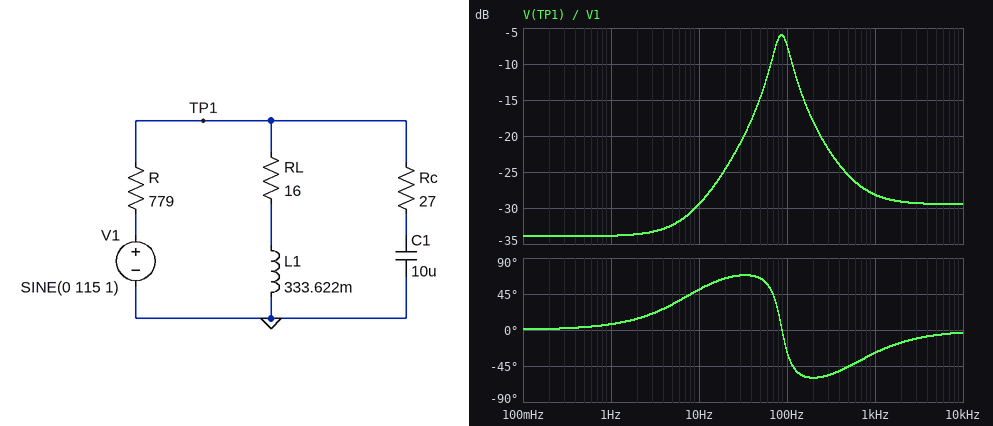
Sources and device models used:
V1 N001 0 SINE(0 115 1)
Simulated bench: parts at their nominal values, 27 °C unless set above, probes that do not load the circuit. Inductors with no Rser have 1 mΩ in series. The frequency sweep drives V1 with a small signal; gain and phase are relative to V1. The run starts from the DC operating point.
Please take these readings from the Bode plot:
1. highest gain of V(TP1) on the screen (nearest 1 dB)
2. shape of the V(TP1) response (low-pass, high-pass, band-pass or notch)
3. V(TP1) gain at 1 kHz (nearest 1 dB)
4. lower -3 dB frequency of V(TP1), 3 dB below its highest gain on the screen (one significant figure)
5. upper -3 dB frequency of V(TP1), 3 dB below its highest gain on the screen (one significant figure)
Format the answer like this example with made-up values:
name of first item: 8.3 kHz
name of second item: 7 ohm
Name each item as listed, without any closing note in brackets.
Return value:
highest gain of V(TP1) on the screen: -6 dB
shape of the V(TP1) response: band-pass
V(TP1) gain at 1 kHz: -28 dB
lower -3 dB frequency of V(TP1), 3 dB below its highest gain on the screen: 70 Hz
upper -3 dB frequency of V(TP1), 3 dB below its highest gain on the screen: 100 Hz
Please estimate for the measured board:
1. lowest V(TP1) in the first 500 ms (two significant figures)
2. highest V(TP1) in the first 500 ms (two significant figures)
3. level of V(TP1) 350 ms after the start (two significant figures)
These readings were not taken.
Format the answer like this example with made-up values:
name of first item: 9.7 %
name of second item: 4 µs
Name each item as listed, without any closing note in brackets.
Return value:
lowest V(TP1) in the first 500 ms: -300 mV
highest V(TP1) in the first 500 ms: 2.3 V
level of V(TP1) 350 ms after the start: 1.7 V
